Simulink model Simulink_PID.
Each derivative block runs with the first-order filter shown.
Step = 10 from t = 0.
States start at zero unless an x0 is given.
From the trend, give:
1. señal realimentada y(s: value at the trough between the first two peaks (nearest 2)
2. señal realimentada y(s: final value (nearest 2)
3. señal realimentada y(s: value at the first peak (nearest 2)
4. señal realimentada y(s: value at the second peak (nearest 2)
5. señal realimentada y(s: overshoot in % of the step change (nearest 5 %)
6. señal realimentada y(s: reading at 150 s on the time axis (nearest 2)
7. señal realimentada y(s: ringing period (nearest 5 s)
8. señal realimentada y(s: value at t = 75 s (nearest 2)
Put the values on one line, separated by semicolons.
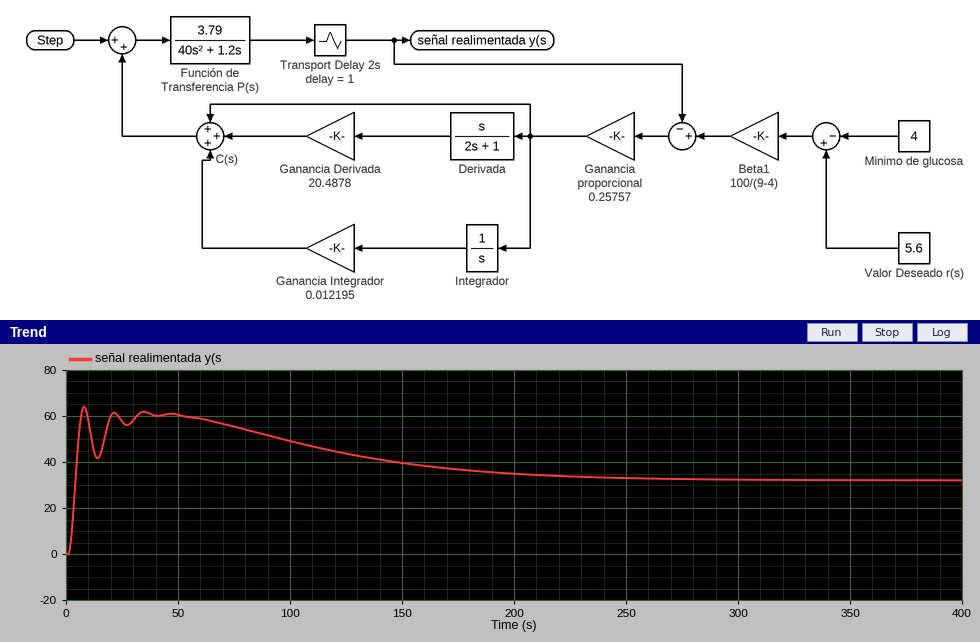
42; 32; 64; 62; 100 %; 40; 15 s; 56
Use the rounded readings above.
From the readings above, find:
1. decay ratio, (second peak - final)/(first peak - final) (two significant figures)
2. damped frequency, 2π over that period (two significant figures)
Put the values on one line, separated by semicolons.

0.94; 0.42 rad/s
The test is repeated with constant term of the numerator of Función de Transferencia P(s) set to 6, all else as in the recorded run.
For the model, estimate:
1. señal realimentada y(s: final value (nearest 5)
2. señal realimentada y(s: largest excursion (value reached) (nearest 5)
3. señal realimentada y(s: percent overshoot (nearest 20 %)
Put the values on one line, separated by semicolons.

30; 75; 140 %
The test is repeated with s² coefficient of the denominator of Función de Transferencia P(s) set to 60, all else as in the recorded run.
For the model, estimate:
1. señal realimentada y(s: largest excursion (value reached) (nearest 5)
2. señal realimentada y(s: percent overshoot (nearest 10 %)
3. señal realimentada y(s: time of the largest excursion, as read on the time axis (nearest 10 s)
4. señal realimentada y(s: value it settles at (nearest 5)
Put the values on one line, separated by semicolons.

60; 90 %; 40 s; 30
